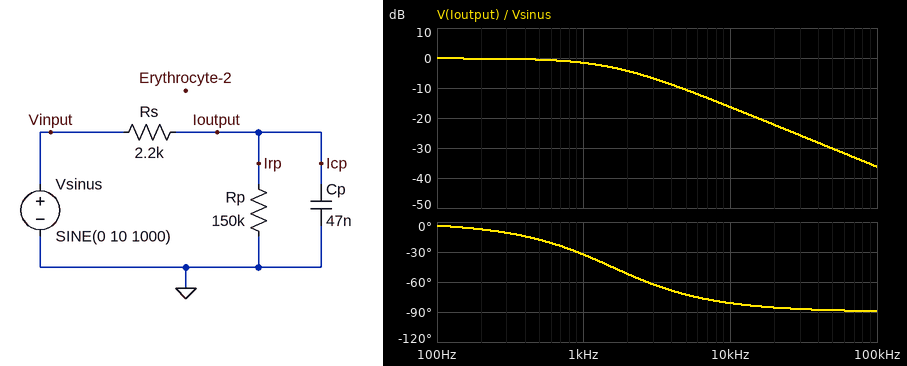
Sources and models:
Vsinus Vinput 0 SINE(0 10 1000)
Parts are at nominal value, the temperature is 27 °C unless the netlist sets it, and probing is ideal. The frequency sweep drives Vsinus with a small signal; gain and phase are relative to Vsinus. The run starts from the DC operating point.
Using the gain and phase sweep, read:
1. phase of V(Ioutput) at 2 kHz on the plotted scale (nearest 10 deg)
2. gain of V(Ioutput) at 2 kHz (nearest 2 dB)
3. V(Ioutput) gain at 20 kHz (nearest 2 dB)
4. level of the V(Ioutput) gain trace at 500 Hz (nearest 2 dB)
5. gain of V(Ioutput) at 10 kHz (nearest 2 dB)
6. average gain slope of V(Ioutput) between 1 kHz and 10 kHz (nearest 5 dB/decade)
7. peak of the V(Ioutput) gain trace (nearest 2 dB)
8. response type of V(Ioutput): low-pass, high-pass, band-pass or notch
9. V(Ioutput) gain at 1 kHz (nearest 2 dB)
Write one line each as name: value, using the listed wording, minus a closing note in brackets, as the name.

phase of V(Ioutput) at 2 kHz on the plotted scale: -50 deg
gain of V(Ioutput) at 2 kHz: -4 dB
V(Ioutput) gain at 20 kHz: -22 dB
level of the V(Ioutput) gain trace at 500 Hz: 0 dB
gain of V(Ioutput) at 10 kHz: -16 dB
average gain slope of V(Ioutput) between 1 kHz and 10 kHz: -15 dB/decade
peak of the V(Ioutput) gain trace: 0 dB
response type of V(Ioutput): low-pass, high-pass, band-pass or notch: low-pass
V(Ioutput) gain at 1 kHz: -2 dB
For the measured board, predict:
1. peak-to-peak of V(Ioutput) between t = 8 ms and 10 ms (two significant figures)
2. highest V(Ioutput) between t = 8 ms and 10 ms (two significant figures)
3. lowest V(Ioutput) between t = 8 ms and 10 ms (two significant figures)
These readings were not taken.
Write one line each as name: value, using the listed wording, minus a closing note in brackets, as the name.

peak-to-peak of V(Ioutput) between t = 8 ms and 10 ms: 17 V
highest V(Ioutput) between t = 8 ms and 10 ms: 8.3 V
lowest V(Ioutput) between t = 8 ms and 10 ms: -8.3 V
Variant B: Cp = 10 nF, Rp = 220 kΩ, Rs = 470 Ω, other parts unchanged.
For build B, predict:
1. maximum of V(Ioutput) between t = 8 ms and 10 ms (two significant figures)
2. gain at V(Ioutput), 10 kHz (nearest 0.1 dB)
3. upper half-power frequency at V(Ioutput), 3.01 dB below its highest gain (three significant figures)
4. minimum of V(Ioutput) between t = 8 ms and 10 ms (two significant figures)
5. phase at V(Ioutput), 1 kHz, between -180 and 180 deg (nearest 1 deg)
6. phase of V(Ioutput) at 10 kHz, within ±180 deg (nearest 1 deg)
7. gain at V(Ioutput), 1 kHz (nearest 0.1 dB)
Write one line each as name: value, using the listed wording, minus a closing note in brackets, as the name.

maximum of V(Ioutput) between t = 8 ms and 10 ms: 10 V
gain at V(Ioutput), 10 kHz: -0.4 dB
upper half-power frequency at V(Ioutput), 3.01 dB below its highest gain: 33.9 kHz
minimum of V(Ioutput) between t = 8 ms and 10 ms: -10 V
phase at V(Ioutput), 1 kHz, between -180 and 180 deg: -2 deg
phase of V(Ioutput) at 10 kHz, within ±180 deg: -16 deg
gain at V(Ioutput), 1 kHz: 0 dB
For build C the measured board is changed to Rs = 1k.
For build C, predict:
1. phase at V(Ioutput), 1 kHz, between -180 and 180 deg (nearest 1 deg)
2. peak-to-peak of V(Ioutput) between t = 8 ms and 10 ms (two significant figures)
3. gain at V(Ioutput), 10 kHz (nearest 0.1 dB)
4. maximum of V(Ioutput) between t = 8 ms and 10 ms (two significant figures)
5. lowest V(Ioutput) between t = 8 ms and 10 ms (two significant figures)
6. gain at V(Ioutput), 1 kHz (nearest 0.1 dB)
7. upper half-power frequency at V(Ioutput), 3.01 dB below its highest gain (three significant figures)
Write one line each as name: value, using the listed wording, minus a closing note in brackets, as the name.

phase at V(Ioutput), 1 kHz, between -180 and 180 deg: -16 deg
peak-to-peak of V(Ioutput) between t = 8 ms and 10 ms: 19 V
gain at V(Ioutput), 10 kHz: -9.9 dB
maximum of V(Ioutput) between t = 8 ms and 10 ms: 9.5 V
lowest V(Ioutput) between t = 8 ms and 10 ms: -9.5 V
gain at V(Ioutput), 1 kHz: -0.4 dB
upper half-power frequency at V(Ioutput), 3.01 dB below its highest gain: 3.41 kHz
